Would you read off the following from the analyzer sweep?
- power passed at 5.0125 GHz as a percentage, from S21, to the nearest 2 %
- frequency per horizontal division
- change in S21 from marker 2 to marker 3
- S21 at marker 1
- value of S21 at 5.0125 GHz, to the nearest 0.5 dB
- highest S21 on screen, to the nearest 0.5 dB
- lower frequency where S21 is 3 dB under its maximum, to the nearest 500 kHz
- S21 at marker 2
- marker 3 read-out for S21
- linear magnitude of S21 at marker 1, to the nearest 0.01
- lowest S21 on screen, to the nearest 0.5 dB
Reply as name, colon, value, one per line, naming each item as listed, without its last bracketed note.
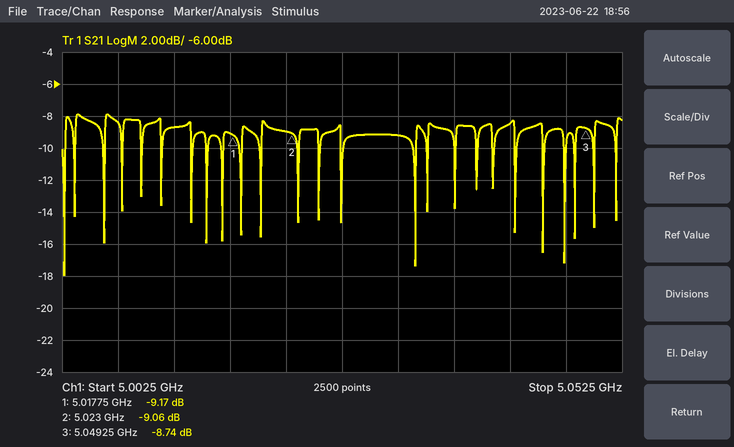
power passed at 5.0125 GHz as a percentage, from S21, to the nearest 2 %: 14 %
frequency per horizontal division: 5 MHz
change in S21 from marker 2 to marker 3: 0.32 dB
S21 at marker 1: -9.17 dB
value of S21 at 5.0125 GHz, to the nearest 0.5 dB: -8.5 dB
highest S21 on screen, to the nearest 0.5 dB: -8.0 dB
lower frequency where S21 is 3 dB under its maximum, to the nearest 500 kHz: 5.0035 GHz
S21 at marker 2: -9.06 dB
marker 3 read-out for S21: -8.74 dB
linear magnitude of S21 at marker 1, to the nearest 0.01: 0.35
lowest S21 on screen, to the nearest 0.5 dB: -18.0 dB
